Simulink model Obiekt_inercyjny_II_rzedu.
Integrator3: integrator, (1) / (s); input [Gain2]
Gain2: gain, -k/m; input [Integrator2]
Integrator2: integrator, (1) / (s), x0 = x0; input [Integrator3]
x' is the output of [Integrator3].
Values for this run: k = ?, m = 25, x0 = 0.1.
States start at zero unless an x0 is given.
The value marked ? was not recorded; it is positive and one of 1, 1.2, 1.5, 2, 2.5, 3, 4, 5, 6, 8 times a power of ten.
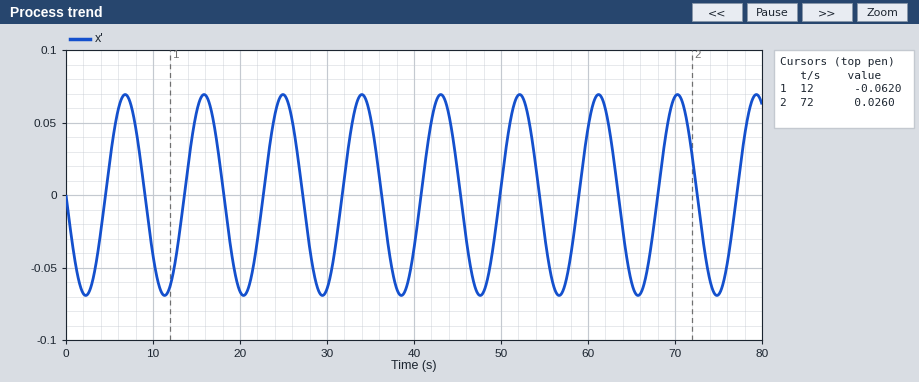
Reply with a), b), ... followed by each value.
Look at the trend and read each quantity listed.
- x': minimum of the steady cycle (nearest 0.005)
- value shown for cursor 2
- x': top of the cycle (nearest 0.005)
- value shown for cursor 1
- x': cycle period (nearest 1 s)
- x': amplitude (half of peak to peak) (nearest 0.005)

a) -0.070
b) 0.0260
c) 0.070
d) -0.0620
e) 9 s
f) 0.070
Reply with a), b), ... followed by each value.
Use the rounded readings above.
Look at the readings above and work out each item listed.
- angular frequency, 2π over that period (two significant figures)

a) 0.70 rad/s
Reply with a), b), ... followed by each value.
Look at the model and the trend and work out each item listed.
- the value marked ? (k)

a) 12
